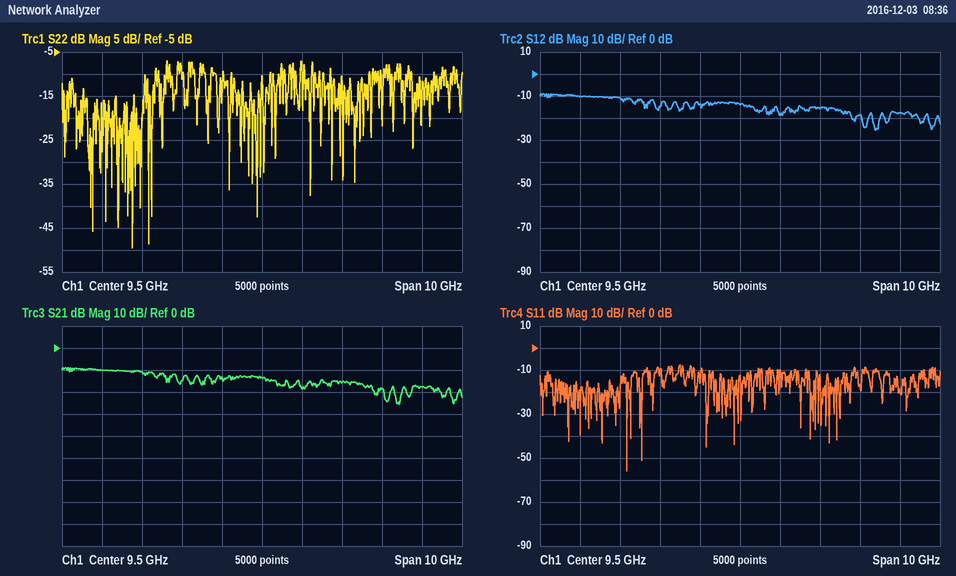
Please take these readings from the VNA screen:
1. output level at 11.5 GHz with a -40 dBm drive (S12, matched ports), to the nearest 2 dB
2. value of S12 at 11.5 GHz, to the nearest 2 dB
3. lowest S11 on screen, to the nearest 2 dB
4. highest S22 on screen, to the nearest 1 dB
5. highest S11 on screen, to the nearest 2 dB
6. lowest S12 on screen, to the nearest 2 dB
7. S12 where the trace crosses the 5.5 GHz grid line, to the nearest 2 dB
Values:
-56 dBm
-16 dB
-56 dB
-7 dB
-8 dB
-26 dB
-10 dB
